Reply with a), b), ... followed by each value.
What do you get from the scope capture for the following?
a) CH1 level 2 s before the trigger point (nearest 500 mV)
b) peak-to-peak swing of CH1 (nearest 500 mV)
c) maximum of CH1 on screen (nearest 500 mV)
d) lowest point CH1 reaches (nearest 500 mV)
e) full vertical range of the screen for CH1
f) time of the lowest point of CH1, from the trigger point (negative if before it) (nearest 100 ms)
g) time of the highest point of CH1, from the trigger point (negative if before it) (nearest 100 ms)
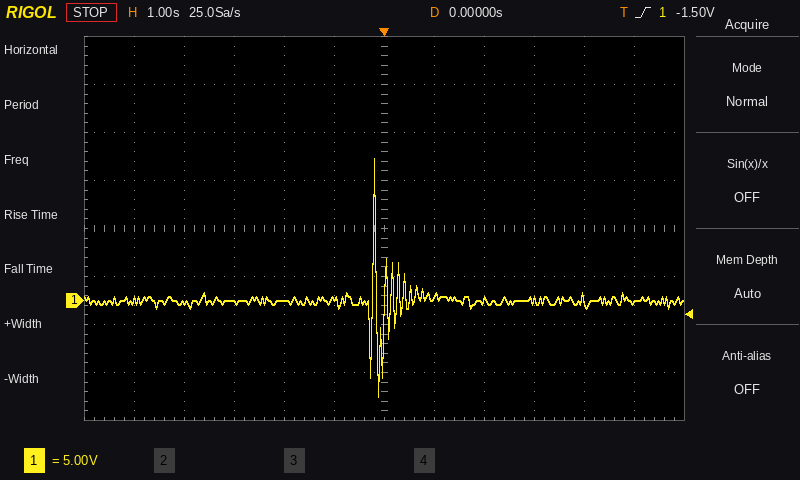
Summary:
a) 0.0 V
b) 25.0 V
c) 15.0 V
d) -10.0 V
e) 40 V
f) -100 ms
g) -200 ms
